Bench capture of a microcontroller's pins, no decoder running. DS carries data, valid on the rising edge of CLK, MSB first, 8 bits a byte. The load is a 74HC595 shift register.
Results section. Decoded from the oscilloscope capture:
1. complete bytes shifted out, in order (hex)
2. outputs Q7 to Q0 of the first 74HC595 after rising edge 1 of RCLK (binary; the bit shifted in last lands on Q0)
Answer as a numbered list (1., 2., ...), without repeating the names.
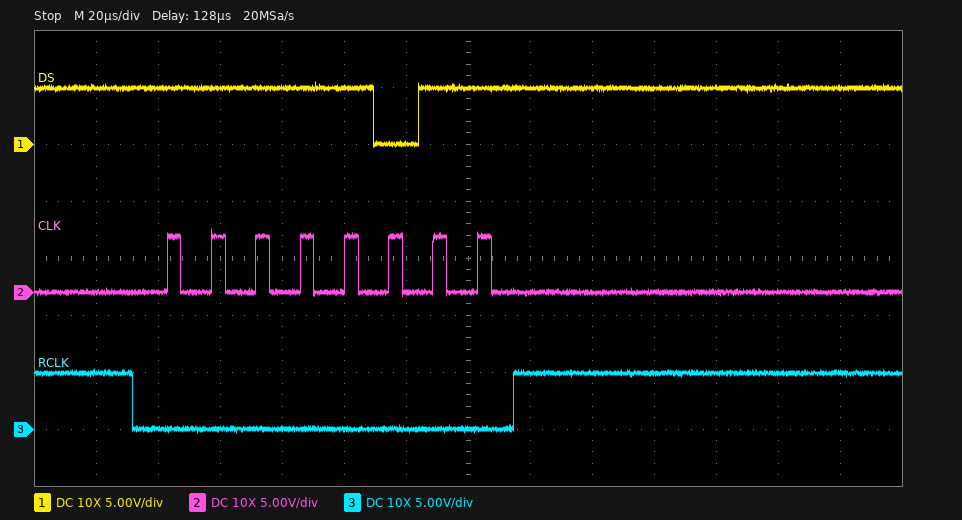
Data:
1. FB
2. 11111011
